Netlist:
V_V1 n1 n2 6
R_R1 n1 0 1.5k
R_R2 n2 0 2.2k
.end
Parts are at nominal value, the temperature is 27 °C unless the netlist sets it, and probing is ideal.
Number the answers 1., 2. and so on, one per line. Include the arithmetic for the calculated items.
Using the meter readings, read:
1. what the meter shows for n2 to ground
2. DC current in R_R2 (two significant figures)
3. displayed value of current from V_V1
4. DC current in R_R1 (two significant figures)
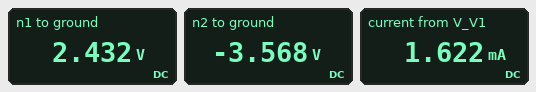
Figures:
1. -3.568 V
2. (0 V - (-3.568 V)) / 2.2 kΩ = 1.6 mA
3. 1.622 mA
4. (2.432 V) / 1.5 kΩ = 1.6 mA
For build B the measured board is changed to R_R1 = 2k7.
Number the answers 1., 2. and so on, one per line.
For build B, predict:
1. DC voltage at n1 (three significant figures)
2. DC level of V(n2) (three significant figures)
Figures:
1. 3.31 V
2. -2.69 V
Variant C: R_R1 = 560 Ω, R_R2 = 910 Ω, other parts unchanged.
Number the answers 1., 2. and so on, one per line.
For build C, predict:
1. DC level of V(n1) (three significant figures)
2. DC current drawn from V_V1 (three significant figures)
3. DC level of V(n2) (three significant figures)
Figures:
1. 2.29 V
2. 4.08 mA
3. -3.71 V
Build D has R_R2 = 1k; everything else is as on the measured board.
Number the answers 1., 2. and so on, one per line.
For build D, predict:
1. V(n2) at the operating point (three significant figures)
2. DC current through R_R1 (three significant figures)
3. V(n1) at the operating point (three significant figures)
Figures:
1. -2.40 V
2. 2.40 mA
3. 3.60 V
